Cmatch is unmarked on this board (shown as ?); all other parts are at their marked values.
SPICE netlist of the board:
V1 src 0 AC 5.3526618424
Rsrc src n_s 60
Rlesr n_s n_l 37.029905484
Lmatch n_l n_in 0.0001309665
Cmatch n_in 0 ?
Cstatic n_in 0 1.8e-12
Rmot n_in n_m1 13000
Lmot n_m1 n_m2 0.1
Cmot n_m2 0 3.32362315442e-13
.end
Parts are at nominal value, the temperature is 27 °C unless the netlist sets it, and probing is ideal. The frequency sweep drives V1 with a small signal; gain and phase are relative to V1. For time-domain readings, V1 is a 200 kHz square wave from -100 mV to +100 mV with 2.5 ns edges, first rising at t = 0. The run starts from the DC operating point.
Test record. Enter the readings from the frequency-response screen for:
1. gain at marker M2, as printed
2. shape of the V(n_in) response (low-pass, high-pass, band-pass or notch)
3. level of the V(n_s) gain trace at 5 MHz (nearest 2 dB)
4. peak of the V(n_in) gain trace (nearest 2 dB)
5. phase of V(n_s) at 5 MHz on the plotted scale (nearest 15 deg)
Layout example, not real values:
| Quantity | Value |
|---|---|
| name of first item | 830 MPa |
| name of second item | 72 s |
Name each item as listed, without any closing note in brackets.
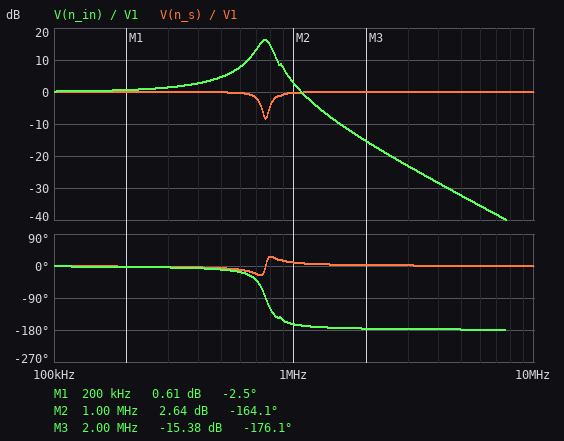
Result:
| Quantity | Value |
|---|---|
| gain at marker M2, as printed | 2.64 dB |
| shape of the V(n_in) response | low-pass |
| level of the V(n_s) gain trace at 5 MHz | 0 dB |
| peak of the V(n_in) gain trace | 16 dB |
| phase of V(n_s) at 5 MHz on the plotted scale | 0 deg |
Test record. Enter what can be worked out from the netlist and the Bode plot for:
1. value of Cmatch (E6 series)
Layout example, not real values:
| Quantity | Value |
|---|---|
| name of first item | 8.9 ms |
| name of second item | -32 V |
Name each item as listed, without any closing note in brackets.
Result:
| Quantity | Value |
|---|---|
| value of Cmatch | 330 pF |
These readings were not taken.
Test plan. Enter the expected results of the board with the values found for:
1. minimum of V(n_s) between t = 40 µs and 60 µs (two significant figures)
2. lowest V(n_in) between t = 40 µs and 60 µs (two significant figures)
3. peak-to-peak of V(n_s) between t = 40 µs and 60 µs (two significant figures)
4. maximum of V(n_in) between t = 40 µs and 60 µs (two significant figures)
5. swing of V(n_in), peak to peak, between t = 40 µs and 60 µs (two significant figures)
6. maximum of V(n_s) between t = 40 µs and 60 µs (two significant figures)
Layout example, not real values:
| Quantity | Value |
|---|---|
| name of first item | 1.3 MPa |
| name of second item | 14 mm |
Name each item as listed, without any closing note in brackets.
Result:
| Quantity | Value |
|---|---|
| minimum of V(n_s) between t = 40 µs and 60 µs | -110 mV |
| lowest V(n_in) between t = 40 µs and 60 µs | -220 mV |
| peak-to-peak of V(n_s) between t = 40 µs and 60 µs | 220 mV |
| maximum of V(n_in) between t = 40 µs and 60 µs | 220 mV |
| swing of V(n_in), peak to peak, between t = 40 µs and 60 µs | 440 mV |
| maximum of V(n_s) between t = 40 µs and 60 µs | 110 mV |
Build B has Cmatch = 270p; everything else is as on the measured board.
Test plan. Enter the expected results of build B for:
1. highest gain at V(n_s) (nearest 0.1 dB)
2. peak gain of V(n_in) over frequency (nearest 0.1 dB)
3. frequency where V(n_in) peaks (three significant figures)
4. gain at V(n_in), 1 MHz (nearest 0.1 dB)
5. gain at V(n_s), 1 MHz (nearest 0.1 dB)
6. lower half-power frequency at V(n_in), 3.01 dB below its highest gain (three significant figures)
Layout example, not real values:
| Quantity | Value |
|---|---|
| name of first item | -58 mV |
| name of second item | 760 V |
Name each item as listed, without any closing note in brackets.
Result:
| Quantity | Value |
|---|---|
| highest gain at V(n_s) | 0 dB |
| peak gain of V(n_in) over frequency | 16.9 dB |
| frequency where V(n_in) peaks | 831 kHz |
| gain at V(n_in), 1 MHz | 7.3 dB |
| gain at V(n_s), 1 MHz | -0.6 dB |
| lower half-power frequency at V(n_in), 3.01 dB below its highest gain | 773 kHz |
